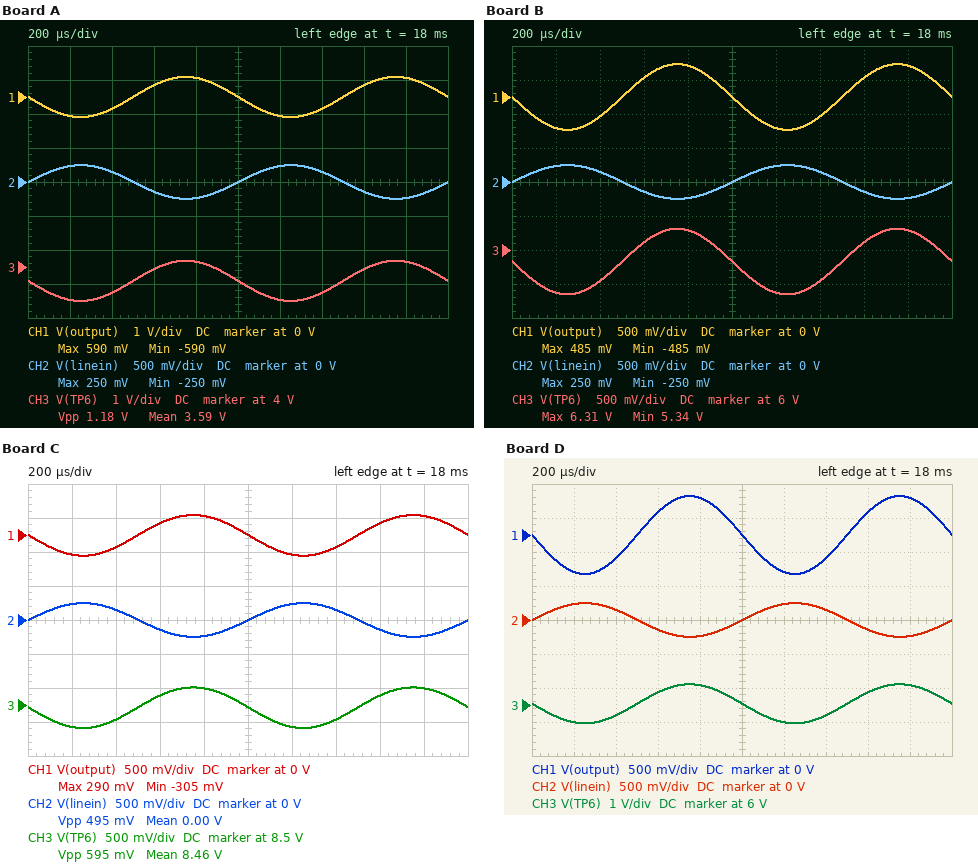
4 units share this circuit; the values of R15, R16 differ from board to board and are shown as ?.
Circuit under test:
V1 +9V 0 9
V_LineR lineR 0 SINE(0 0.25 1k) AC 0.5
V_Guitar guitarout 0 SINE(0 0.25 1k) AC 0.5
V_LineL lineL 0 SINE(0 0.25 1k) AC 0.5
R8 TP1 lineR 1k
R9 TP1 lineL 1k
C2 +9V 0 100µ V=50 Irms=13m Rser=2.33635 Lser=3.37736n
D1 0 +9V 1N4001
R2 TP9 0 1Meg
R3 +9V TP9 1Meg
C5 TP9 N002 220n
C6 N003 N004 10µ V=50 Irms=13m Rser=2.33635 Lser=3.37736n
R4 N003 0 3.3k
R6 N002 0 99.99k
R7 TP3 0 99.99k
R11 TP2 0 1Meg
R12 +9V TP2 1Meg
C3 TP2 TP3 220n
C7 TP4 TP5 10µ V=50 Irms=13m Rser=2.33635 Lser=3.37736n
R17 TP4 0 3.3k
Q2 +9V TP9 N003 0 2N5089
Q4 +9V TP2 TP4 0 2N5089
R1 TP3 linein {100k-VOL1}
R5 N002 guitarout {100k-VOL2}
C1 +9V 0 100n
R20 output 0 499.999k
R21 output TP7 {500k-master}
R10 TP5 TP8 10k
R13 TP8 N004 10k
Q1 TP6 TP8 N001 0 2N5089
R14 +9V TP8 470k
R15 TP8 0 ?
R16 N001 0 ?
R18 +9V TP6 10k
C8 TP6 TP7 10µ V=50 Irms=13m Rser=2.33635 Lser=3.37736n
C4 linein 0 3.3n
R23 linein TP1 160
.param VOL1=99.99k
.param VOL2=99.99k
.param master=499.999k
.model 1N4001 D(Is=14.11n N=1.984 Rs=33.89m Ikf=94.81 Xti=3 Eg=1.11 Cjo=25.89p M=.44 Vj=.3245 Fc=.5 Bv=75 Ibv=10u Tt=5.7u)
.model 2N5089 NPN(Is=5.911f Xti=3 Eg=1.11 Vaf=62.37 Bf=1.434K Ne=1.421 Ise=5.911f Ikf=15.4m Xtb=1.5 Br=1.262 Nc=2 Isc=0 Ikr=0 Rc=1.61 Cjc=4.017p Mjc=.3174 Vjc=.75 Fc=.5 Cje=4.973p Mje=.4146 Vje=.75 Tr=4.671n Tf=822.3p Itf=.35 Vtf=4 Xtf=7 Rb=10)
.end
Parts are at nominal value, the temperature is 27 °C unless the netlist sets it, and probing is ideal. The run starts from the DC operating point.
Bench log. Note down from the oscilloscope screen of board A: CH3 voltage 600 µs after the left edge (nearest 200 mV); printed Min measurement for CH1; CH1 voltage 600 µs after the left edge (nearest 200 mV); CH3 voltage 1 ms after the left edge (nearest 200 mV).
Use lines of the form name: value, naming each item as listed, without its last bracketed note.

CH3 voltage 600 µs after the left edge: 4.0 V
printed Min measurement for CH1: -590 mV
CH1 voltage 600 µs after the left edge: 400 mV
CH3 voltage 1 ms after the left edge: 3.6 V
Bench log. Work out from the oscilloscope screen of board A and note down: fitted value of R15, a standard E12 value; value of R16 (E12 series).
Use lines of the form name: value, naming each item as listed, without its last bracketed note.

fitted value of R15, a standard E12 value: 220 kΩ
value of R16: 3.9 kΩ
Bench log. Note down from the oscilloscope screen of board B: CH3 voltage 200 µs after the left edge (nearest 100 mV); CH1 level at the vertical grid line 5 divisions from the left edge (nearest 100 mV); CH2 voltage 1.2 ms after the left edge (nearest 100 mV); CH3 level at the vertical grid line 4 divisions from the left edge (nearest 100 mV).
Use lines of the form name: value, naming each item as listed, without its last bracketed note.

CH3 voltage 200 µs after the left edge: 5.4 V
CH1 level at the vertical grid line 5 divisions from the left edge: 0 V
CH2 voltage 1.2 ms after the left edge: 200 mV
CH3 level at the vertical grid line 4 divisions from the left edge: 6.3 V
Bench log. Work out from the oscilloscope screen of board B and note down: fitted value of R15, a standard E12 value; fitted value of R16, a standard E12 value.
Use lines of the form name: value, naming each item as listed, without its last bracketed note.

fitted value of R15, a standard E12 value: 150 kΩ
fitted value of R16, a standard E12 value: 4.7 kΩ
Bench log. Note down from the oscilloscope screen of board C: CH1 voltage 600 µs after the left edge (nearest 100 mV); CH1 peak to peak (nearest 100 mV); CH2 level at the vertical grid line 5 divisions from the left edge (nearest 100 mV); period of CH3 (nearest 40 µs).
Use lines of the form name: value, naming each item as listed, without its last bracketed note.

CH1 voltage 600 µs after the left edge: 200 mV
CH1 peak to peak: 600 mV
CH2 level at the vertical grid line 5 divisions from the left edge: 0 V
period of CH3: 1.00 ms
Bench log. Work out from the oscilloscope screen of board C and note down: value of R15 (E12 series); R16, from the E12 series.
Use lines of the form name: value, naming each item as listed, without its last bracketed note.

value of R15: 56 kΩ
R16, from the E12 series: 6.8 kΩ
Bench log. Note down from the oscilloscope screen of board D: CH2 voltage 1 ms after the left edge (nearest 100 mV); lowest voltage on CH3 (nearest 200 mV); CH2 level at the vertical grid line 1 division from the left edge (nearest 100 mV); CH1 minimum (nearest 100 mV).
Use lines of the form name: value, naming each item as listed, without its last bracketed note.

CH2 voltage 1 ms after the left edge: 0 V
lowest voltage on CH3: 5.4 V
CH2 level at the vertical grid line 1 division from the left edge: 200 mV
CH1 minimum: -600 mV
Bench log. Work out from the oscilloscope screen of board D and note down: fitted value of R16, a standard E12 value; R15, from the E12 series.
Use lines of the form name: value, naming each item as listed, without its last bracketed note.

fitted value of R16, a standard E12 value: 3.9 kΩ
R15, from the E12 series: 120 kΩ
